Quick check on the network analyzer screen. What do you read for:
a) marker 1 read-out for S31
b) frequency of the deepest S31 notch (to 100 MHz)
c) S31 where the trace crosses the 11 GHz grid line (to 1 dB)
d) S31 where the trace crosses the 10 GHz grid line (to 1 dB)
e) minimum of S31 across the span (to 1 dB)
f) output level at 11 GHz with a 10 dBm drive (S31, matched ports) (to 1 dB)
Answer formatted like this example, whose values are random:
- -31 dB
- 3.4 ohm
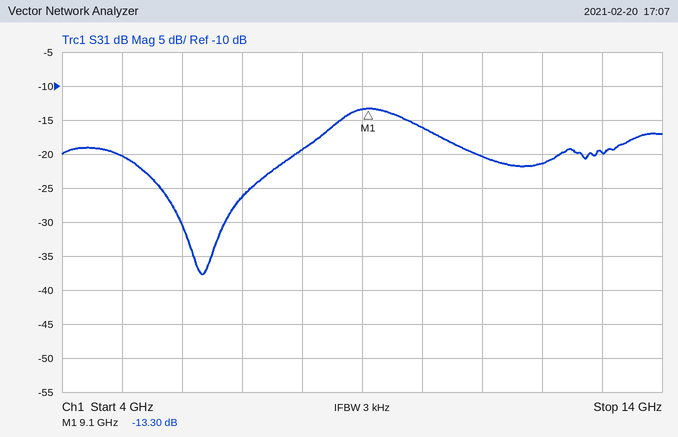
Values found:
- -13.30 dB
- 6.3 GHz
- -20 dB
- -16 dB
- -38 dB
- -10 dBm
